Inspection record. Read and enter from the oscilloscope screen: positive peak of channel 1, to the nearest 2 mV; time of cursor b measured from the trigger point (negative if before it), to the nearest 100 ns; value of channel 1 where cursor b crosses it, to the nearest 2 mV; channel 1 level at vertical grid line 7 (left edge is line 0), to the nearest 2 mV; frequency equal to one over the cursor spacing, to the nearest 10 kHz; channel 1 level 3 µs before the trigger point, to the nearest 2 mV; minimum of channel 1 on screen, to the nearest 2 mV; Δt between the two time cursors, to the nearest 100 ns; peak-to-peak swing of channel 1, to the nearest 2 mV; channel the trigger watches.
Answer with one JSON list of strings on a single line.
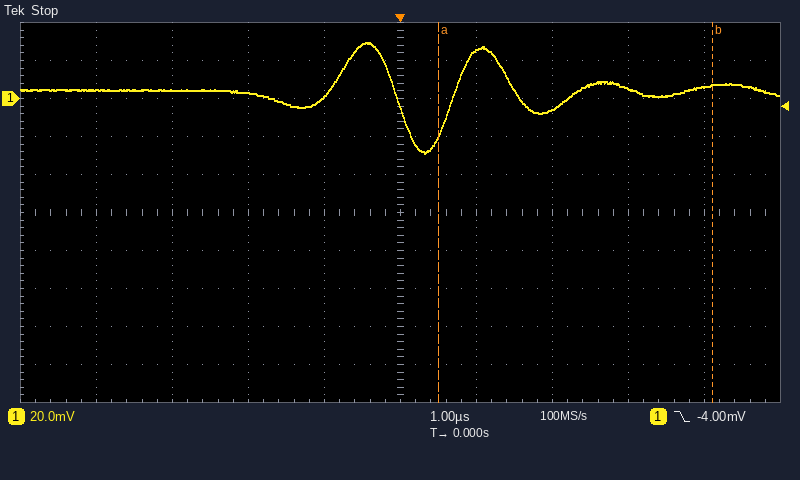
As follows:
["30 mV", "+4.1 µs", "6 mV", "-6 mV", "280 kHz", "4 mV", "-28 mV", "3.6 µs", "58 mV", "channel 1"]
